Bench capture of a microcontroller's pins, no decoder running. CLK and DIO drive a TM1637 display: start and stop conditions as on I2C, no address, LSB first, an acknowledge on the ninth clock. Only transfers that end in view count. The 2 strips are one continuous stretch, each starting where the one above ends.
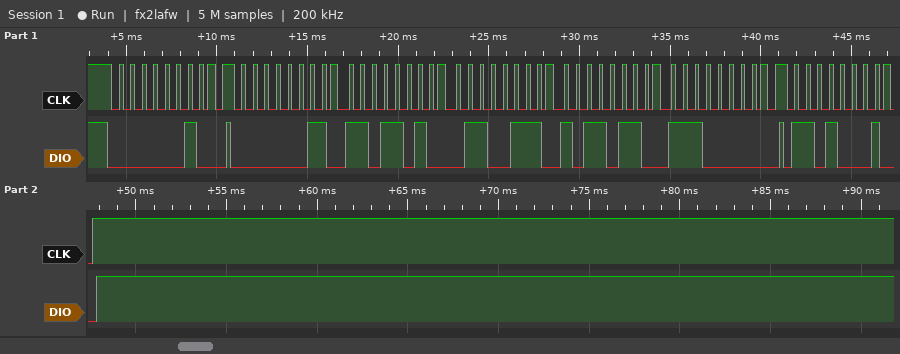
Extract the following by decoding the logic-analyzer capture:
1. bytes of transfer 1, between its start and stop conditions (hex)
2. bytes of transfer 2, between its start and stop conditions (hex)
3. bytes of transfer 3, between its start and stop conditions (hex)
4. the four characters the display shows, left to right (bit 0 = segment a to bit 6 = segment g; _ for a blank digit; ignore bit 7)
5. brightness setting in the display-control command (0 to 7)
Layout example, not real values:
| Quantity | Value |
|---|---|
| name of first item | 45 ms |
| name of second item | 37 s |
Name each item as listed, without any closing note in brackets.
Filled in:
| Quantity | Value |
|---|---|
| bytes of transfer 1, between its start and stop conditions | 40 |
| bytes of transfer 2, between its start and stop conditions | C0 5B E6 6D 07 |
| bytes of transfer 3, between its start and stop conditions | 8B |
| the four characters the display shows, left to right | 2457 |
| brightness setting in the display-control command | 3 |
